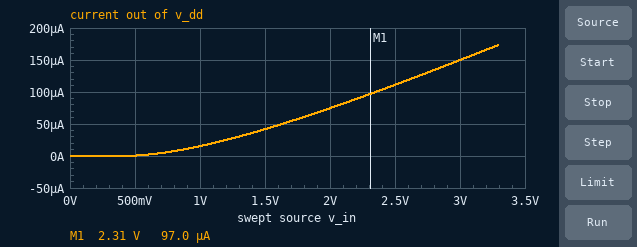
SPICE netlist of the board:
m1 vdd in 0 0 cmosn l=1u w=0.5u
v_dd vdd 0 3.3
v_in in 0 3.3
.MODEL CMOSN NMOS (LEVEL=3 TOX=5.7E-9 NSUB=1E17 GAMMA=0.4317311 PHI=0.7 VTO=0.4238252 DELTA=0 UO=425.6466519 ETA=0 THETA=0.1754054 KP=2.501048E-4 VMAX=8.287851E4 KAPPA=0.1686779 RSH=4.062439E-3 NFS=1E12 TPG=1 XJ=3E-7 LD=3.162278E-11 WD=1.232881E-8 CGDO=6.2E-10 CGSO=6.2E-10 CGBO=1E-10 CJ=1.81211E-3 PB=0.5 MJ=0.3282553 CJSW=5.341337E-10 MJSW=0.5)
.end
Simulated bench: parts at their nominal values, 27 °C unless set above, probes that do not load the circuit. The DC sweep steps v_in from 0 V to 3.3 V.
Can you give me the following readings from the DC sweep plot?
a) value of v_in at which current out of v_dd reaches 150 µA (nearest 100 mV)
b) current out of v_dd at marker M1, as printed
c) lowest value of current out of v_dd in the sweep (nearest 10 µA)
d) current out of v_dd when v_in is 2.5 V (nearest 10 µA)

3.0 V
97.0 µA
0 A
110 µA
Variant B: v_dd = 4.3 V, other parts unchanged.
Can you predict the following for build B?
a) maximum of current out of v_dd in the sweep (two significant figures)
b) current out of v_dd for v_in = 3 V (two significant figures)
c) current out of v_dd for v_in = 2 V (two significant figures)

180 µA
150 µA
76 µA
